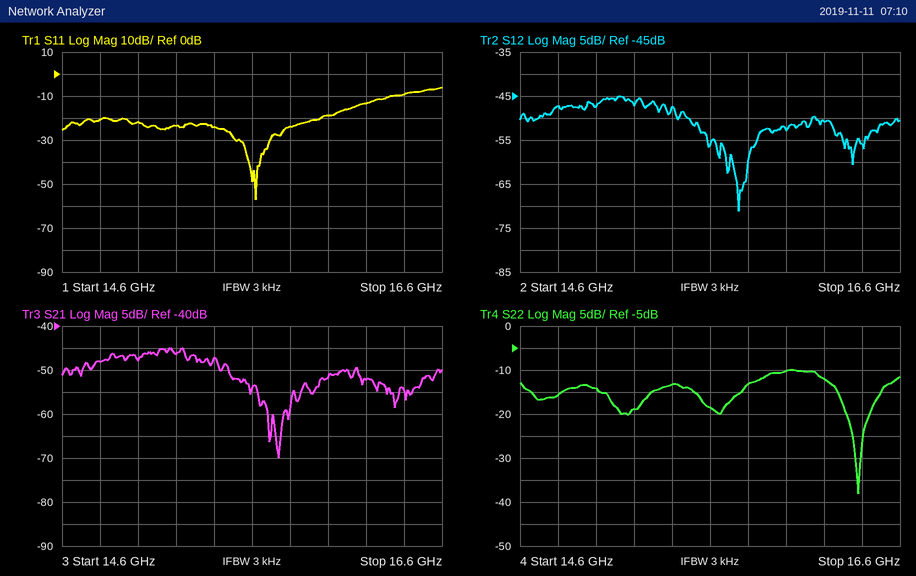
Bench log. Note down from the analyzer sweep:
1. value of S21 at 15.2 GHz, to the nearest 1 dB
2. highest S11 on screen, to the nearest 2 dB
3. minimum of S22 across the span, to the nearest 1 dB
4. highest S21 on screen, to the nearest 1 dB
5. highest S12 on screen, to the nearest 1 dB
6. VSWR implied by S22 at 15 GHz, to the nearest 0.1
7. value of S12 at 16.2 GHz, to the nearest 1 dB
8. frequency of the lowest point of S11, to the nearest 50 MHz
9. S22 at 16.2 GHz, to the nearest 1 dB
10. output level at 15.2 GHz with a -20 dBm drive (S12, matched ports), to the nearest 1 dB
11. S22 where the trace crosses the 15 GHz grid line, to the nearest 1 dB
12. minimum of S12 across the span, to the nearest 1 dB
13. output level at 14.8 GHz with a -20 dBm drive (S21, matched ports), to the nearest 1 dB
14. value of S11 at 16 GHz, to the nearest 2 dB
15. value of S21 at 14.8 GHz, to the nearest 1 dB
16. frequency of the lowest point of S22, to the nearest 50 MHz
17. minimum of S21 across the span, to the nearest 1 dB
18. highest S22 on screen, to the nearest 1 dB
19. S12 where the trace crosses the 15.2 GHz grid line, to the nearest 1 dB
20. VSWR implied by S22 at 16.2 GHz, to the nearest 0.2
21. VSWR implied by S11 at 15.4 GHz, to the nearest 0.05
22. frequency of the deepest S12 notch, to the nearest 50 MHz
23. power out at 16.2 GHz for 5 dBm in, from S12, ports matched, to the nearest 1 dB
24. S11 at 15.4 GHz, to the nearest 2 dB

-46 dB
-6 dB
-38 dB
-45 dB
-45 dB
1.5
-51 dB
15.60 GHz
-12 dB
-67 dBm
-14 dB
-71 dB
-68 dBm
-18 dB
-48 dB
16.40 GHz
-70 dB
-10 dB
-47 dB
1.6
1.15
15.75 GHz
-46 dBm
-24 dB
